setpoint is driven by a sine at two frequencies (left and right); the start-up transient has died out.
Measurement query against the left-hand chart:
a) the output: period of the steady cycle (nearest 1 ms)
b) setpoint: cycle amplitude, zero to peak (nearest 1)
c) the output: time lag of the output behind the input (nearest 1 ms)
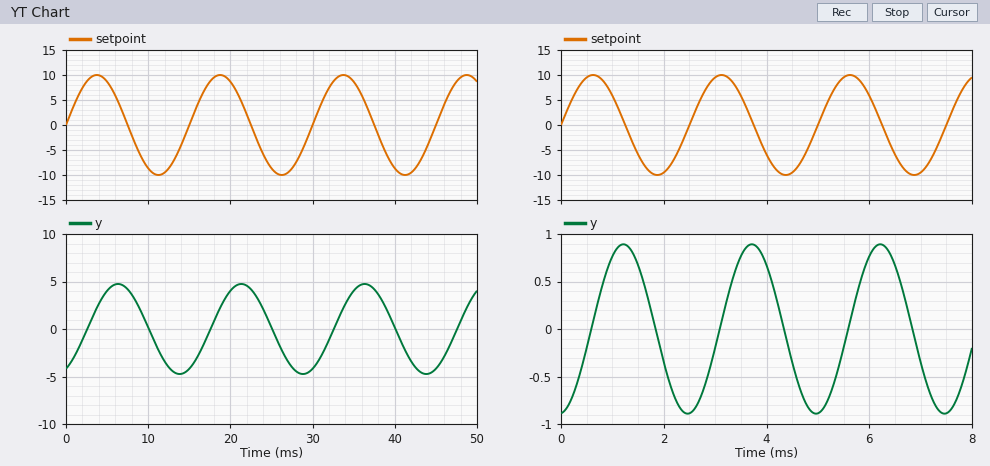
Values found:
15 ms
10
3 ms
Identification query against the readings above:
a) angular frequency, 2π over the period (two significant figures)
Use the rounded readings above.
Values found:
0.42 rad/ms
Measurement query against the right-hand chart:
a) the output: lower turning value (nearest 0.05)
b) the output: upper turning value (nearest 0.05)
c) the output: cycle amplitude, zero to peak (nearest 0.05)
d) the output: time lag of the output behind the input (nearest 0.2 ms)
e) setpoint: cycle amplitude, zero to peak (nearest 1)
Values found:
-0.90
0.90
0.90
0.6 ms
10
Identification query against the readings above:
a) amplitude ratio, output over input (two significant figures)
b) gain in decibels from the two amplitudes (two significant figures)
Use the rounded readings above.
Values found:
0.090
-21 dB
